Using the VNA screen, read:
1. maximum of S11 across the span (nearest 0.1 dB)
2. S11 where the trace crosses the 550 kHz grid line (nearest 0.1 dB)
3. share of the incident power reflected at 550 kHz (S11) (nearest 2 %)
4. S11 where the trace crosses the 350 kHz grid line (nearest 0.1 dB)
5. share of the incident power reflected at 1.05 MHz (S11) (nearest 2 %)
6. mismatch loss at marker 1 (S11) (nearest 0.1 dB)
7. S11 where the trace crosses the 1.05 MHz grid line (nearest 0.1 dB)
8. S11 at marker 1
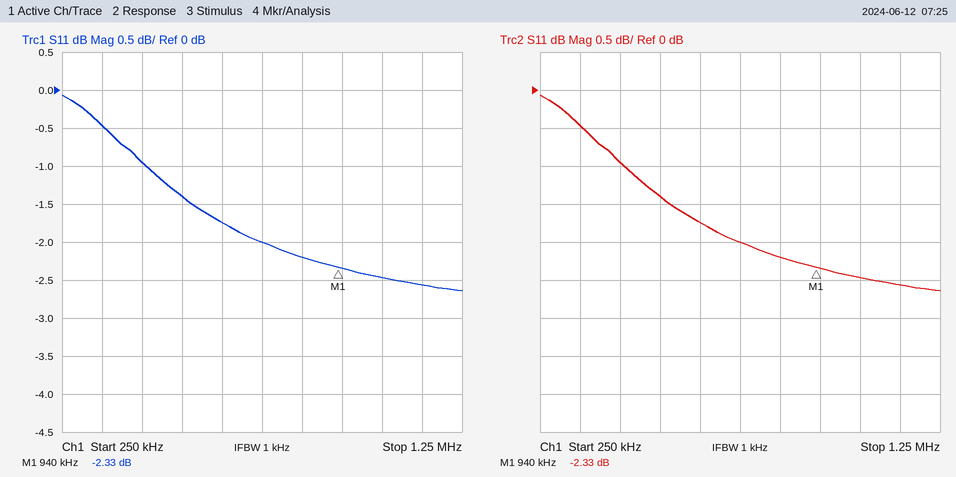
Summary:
-0.1 dB
-1.4 dB
72 %
-0.5 dB
56 %
3.8 dB
-2.5 dB
-2.33 dB
